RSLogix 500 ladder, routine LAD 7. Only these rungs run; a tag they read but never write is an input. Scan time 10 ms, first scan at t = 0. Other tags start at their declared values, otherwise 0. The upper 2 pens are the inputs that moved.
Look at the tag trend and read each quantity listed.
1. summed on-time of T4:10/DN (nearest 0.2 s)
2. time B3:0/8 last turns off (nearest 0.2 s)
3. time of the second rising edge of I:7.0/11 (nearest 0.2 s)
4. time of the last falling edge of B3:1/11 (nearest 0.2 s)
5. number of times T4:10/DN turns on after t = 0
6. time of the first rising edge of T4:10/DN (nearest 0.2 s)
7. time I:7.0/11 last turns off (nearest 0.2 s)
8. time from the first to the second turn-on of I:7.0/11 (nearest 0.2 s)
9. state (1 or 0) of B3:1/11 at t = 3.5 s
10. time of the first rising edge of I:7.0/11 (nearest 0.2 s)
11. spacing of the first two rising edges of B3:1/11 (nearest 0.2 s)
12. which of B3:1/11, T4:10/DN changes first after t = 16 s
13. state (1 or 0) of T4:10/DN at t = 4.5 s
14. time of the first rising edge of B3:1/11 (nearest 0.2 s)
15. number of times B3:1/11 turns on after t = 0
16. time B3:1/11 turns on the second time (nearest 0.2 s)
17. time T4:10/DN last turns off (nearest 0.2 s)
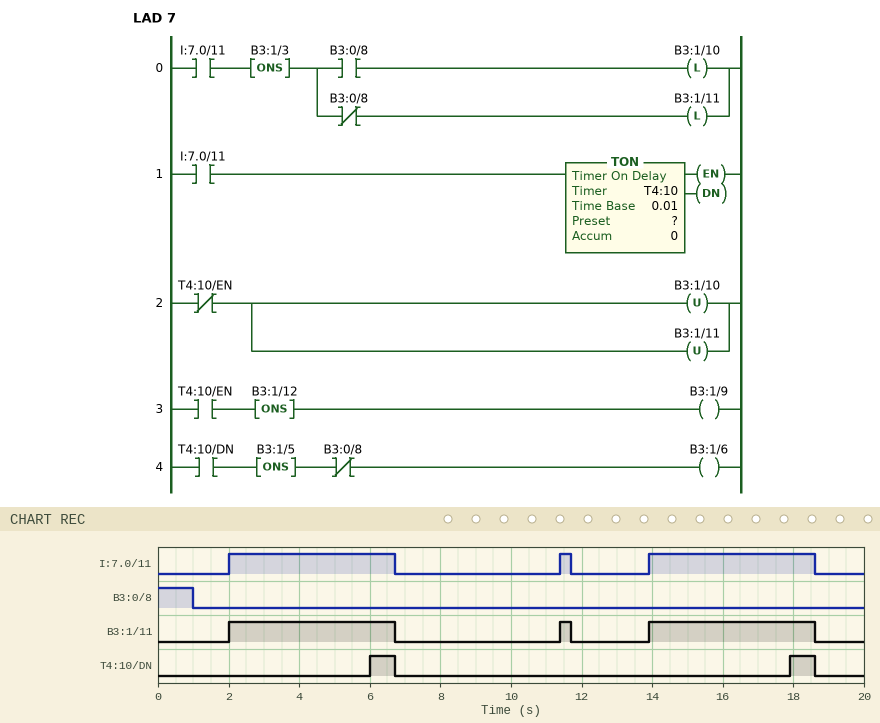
1.4 s
1.0 s
11.4 s
18.6 s
2
6.0 s
18.6 s
9.4 s
1
2.0 s
9.4 s
T4:10/DN
0
2.0 s
3
11.4 s
18.6 s
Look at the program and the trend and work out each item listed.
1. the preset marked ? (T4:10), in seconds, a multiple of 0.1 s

4.0 s
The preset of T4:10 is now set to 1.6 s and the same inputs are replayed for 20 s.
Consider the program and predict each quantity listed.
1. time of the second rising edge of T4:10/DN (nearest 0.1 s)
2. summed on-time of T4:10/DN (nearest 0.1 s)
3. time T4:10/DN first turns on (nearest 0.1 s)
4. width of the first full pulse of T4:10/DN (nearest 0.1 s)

15.5 s
6.2 s
3.6 s
3.1 s
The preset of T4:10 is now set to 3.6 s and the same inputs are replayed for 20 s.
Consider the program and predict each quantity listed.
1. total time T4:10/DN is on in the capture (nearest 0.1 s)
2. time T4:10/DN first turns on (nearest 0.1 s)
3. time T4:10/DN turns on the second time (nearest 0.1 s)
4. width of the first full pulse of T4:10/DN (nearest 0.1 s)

2.2 s
5.6 s
17.5 s
1.1 s
